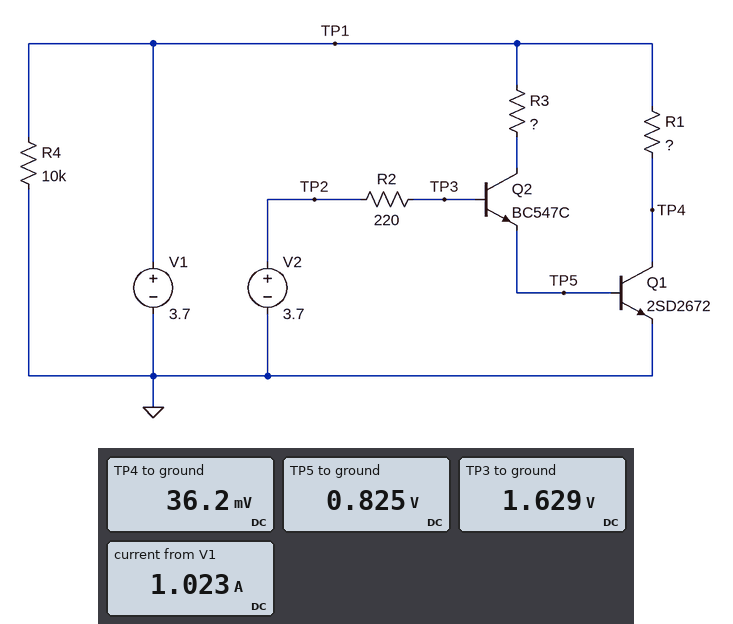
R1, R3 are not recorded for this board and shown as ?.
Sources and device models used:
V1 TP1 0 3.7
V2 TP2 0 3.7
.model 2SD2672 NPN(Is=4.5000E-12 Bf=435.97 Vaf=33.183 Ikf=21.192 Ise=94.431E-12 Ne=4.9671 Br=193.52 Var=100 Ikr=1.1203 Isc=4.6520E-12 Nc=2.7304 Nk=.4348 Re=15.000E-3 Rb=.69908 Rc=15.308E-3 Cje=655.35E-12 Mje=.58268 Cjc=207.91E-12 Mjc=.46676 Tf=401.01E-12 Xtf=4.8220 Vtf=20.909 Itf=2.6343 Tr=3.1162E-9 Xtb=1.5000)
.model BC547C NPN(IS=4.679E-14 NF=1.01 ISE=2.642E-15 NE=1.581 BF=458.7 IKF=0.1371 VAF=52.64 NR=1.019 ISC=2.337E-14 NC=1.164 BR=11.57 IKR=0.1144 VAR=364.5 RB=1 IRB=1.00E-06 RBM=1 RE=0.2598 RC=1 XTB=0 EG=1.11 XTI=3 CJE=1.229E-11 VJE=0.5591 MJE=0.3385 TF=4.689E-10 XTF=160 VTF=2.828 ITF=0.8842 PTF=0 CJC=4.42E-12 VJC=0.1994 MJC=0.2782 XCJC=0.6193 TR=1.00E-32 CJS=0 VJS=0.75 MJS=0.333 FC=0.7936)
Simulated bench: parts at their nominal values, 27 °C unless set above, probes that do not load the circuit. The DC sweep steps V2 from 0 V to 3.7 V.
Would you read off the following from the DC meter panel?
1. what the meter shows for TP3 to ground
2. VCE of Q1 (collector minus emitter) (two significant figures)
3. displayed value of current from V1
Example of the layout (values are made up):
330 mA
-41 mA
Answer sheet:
1.629 V
36 mV
1.023 A
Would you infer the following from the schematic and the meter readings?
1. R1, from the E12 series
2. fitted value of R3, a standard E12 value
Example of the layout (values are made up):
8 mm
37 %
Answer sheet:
3.9 Ω
33 Ω
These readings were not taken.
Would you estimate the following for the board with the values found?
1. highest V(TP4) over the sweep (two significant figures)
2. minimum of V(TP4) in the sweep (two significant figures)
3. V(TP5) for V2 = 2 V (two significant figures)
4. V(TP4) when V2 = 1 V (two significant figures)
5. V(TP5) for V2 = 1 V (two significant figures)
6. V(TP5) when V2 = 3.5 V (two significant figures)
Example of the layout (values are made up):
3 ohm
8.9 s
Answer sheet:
3.7 V
36 mV
820 mV
3.7 V
520 mV
820 mV
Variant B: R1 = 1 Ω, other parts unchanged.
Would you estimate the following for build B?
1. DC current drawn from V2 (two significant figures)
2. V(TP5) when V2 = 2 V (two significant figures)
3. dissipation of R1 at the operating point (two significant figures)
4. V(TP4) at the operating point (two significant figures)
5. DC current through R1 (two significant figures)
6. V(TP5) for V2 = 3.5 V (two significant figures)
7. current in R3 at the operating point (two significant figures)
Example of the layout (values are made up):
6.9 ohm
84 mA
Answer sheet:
9.2 mA
860 mV
13 W
130 mV
3.6 A
870 mV
82 mA
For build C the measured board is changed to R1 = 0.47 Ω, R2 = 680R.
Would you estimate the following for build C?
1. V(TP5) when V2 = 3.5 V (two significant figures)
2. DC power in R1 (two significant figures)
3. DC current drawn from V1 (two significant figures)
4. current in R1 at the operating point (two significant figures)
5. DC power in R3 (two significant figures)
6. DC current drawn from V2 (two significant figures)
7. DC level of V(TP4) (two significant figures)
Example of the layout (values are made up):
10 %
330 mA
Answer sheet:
930 mV
25 W
7.4 A
7.3 A
210 mW
2.9 mA
260 mV
